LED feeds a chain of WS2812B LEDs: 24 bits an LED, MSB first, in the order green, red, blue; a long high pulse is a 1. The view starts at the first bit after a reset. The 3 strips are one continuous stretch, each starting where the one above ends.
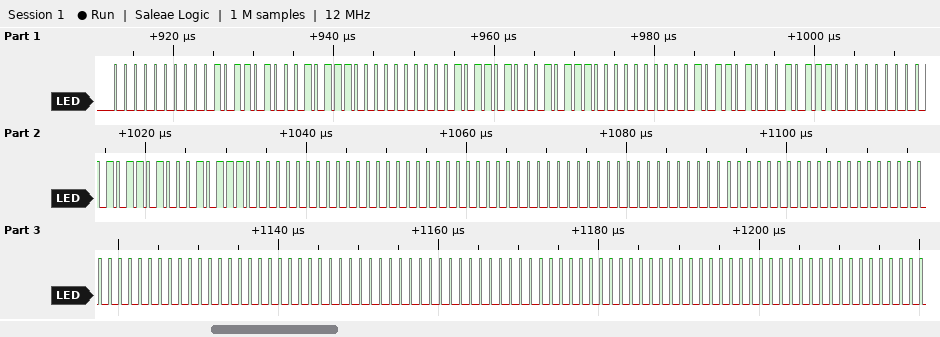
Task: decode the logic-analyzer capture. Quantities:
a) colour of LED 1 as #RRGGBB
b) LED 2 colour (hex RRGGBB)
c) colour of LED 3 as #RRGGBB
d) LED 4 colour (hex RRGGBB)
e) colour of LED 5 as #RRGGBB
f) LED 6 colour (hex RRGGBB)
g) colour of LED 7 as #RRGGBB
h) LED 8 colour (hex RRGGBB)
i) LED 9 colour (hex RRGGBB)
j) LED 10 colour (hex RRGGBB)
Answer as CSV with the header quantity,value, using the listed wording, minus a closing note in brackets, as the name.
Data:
quantity,value
colour of LED 1 as #RRGGBB,#2D0017
LED 2 colour,#2D0017
colour of LED 3 as #RRGGBB,#2D0017
LED 4 colour,#2D0017
colour of LED 5 as #RRGGBB,#000000
LED 6 colour,#000000
colour of LED 7 as #RRGGBB,#000000
LED 8 colour,#000000
LED 9 colour,#000000
LED 10 colour,#000000
